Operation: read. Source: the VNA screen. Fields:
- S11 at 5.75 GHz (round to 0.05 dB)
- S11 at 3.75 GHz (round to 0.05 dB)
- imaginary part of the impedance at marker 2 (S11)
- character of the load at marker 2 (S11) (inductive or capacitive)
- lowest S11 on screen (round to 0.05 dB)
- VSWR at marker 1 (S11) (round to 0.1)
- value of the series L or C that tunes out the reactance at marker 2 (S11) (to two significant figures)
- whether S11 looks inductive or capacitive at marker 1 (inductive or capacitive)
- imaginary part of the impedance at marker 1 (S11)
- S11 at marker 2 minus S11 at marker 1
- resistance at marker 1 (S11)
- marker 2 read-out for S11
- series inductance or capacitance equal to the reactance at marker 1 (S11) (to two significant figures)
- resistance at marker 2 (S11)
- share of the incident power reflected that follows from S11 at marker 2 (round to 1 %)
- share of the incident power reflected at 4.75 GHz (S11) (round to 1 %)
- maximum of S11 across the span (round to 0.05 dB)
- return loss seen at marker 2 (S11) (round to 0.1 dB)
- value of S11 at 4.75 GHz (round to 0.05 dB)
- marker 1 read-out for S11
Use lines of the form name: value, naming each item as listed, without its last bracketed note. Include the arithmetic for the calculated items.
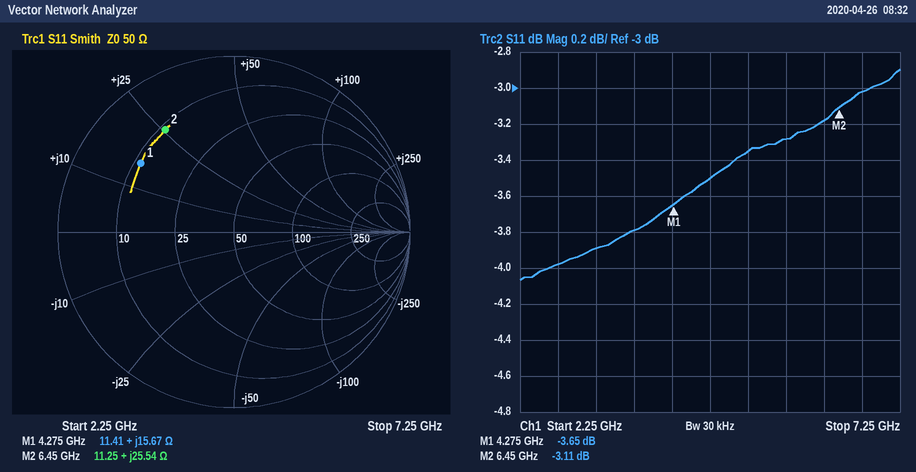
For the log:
S11 at 5.75 GHz: -3.30 dB
S11 at 3.75 GHz: -3.80 dB
imaginary part of the impedance at marker 2: +25.54 Ω
character of the load at marker 2 (S11): inductive
lowest S11 on screen: -4.05 dB
VSWR at marker 1 (S11): 4.8
value of the series L or C that tunes out the reactance at marker 2 (S11): C = 1/(2π × 6.45 GHz × 25.54 Ω) ≈ 966 fF, so 970 fF to two significant figures
whether S11 looks inductive or capacitive at marker 1: inductive
imaginary part of the impedance at marker 1: +15.67 Ω
S11 at marker 2 minus S11 at marker 1: -3.11 − (-3.65) = 0.54 dB
resistance at marker 1: 11.41 Ω
marker 2 read-out for S11: -3.11 dB
series inductance or capacitance equal to the reactance at marker 1 (S11): L = 15.67 Ω/(2π × 4.275 GHz) ≈ 583 pH, so 580 pH to two significant figures
resistance at marker 2: 11.25 Ω
share of the incident power reflected that follows from S11 at marker 2: 10^(-3.11/10) ≈ 49 %
share of the incident power reflected at 4.75 GHz (S11): 10^(-3.5/10) ≈ 45 %
maximum of S11 across the span: -2.90 dB
return loss seen at marker 2 (S11): 3.1 dB
value of S11 at 4.75 GHz: -3.50 dB
marker 1 read-out for S11: -3.65 dB
